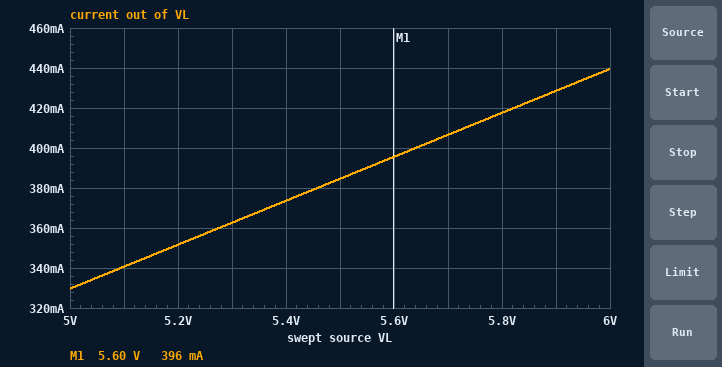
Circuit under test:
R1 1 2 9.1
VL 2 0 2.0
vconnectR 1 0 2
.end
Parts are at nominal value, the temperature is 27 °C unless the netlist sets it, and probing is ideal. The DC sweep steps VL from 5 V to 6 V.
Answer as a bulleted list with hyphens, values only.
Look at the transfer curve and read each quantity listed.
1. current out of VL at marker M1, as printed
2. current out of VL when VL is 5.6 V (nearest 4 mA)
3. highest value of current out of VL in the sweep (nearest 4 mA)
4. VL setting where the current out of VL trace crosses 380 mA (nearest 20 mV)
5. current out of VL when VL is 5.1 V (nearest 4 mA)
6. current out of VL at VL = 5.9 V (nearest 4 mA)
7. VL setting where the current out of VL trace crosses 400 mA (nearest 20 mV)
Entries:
- 396 mA
- 396 mA
- 440 mA
- 5.46 V
- 340 mA
- 428 mA
- 5.64 V
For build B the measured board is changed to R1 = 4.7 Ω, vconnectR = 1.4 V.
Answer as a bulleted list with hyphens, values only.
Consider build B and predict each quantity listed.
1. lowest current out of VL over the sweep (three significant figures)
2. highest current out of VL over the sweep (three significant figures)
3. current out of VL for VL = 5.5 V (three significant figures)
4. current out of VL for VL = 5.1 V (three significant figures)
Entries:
- 766 mA
- 979 mA
- 872 mA
- 787 mA
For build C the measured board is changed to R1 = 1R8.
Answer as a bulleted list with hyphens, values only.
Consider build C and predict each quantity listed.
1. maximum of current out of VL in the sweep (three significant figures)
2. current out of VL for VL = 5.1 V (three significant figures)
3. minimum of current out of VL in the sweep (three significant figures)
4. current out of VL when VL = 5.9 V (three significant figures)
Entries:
- 2.22 A
- 1.72 A
- 1.67 A
- 2.17 A
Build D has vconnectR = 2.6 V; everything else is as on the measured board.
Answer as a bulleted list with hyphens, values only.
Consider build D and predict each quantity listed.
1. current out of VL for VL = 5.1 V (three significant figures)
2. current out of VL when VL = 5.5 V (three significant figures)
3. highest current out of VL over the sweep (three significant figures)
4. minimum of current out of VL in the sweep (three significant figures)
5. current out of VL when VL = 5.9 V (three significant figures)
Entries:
- 275 mA
- 319 mA
- 374 mA
- 264 mA
- 363 mA
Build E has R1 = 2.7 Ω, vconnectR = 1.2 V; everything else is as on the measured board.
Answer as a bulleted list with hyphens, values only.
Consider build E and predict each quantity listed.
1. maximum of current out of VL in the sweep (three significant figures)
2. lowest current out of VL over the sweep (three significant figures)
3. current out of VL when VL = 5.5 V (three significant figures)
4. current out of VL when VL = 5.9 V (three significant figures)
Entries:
- 1.78 A
- 1.41 A
- 1.59 A
- 1.74 A
